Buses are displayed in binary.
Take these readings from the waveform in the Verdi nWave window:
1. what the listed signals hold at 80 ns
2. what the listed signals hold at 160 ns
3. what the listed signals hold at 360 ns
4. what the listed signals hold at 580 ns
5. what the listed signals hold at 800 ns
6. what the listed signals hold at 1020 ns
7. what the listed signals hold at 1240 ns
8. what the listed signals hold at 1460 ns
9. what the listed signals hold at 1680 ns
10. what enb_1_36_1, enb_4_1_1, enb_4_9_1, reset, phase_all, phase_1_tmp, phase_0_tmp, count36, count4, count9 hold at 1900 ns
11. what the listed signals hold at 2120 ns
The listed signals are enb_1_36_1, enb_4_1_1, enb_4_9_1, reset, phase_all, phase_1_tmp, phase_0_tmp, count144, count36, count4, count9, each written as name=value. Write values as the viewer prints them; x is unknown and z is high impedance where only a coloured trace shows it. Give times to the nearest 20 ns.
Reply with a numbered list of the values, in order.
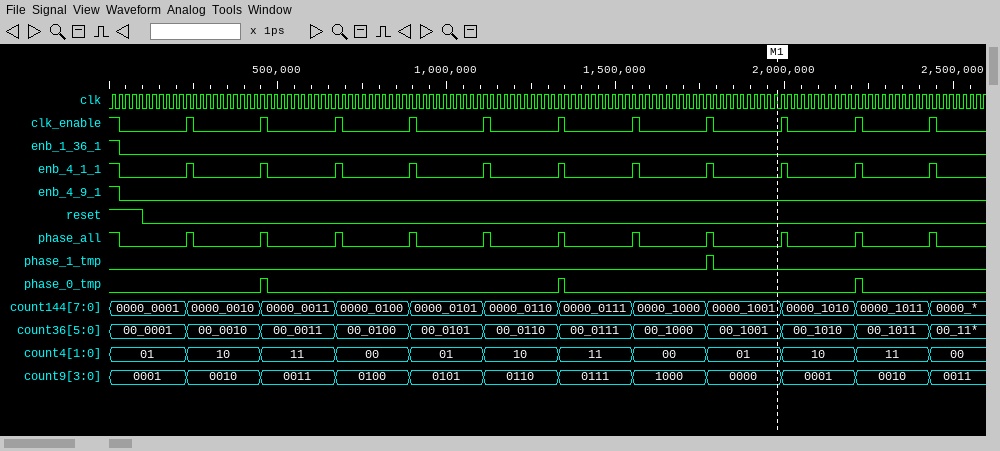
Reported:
1. enb_1_36_1=0, enb_4_1_1=0, enb_4_9_1=0, reset=1, phase_all=0, phase_1_tmp=0, phase_0_tmp=0, count144=0000_0001, count36=00_0001, count4=01, count9=0001
2. enb_1_36_1=0, enb_4_1_1=0, enb_4_9_1=0, reset=0, phase_all=0, phase_1_tmp=0, phase_0_tmp=0, count144=0000_0001, count36=00_0001, count4=01, count9=0001
3. enb_1_36_1=0, enb_4_1_1=0, enb_4_9_1=0, reset=0, phase_all=0, phase_1_tmp=0, phase_0_tmp=0, count144=0000_0010, count36=00_0010, count4=10, count9=0010
4. enb_1_36_1=0, enb_4_1_1=0, enb_4_9_1=0, reset=0, phase_all=0, phase_1_tmp=0, phase_0_tmp=0, count144=0000_0011, count36=00_0011, count4=11, count9=0011
5. enb_1_36_1=0, enb_4_1_1=0, enb_4_9_1=0, reset=0, phase_all=0, phase_1_tmp=0, phase_0_tmp=0, count144=0000_0100, count36=00_0100, count4=00, count9=0100
6. enb_1_36_1=0, enb_4_1_1=0, enb_4_9_1=0, reset=0, phase_all=0, phase_1_tmp=0, phase_0_tmp=0, count144=0000_0101, count36=00_0101, count4=01, count9=0101
7. enb_1_36_1=0, enb_4_1_1=0, enb_4_9_1=0, reset=0, phase_all=0, phase_1_tmp=0, phase_0_tmp=0, count144=0000_0110, count36=00_0110, count4=10, count9=0110
8. enb_1_36_1=0, enb_4_1_1=0, enb_4_9_1=0, reset=0, phase_all=0, phase_1_tmp=0, phase_0_tmp=0, count144=0000_0111, count36=00_0111, count4=11, count9=0111
9. enb_1_36_1=0, enb_4_1_1=0, enb_4_9_1=0, reset=0, phase_all=0, phase_1_tmp=0, phase_0_tmp=0, count144=0000_1000, count36=00_1000, count4=00, count9=1000
10. enb_1_36_1=0, enb_4_1_1=0, enb_4_9_1=0, reset=0, phase_all=0, phase_1_tmp=0, phase_0_tmp=0, count36=00_1001, count4=01, count9=0000
11. enb_1_36_1=0, enb_4_1_1=0, enb_4_9_1=0, reset=0, phase_all=0, phase_1_tmp=0, phase_0_tmp=0, count144=0000_1010, count36=00_1010, count4=10, count9=0001
